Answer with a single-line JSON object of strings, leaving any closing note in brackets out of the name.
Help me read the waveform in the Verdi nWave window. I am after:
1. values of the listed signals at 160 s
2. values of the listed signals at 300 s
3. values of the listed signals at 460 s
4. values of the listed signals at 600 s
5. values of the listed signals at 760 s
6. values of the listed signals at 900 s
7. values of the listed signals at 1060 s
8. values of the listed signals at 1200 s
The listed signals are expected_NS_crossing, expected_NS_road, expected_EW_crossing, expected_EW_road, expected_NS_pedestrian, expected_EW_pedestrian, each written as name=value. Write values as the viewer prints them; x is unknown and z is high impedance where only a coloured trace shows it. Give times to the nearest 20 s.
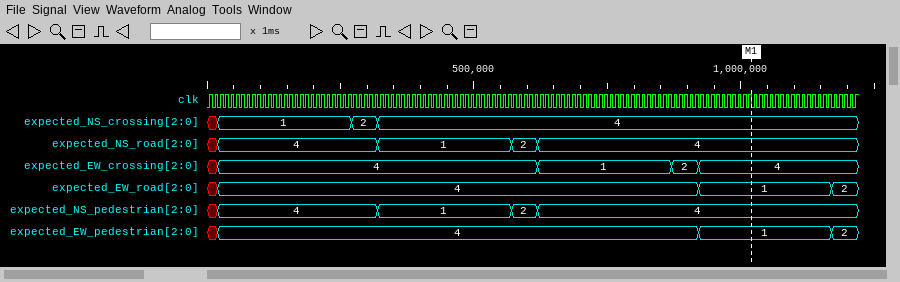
{"values of the listed signals at 160 s": "expected_NS_crossing=1, expected_NS_road=4, expected_EW_crossing=4, expected_EW_road=4, expected_NS_pedestrian=4, expected_EW_pedestrian=4", "values of the listed signals at 300 s": "expected_NS_crossing=2, expected_NS_road=4, expected_EW_crossing=4, expected_EW_road=4, expected_NS_pedestrian=4, expected_EW_pedestrian=4", "values of the listed signals at 460 s": "expected_NS_crossing=4, expected_NS_road=1, expected_EW_crossing=4, expected_EW_road=4, expected_NS_pedestrian=1, expected_EW_pedestrian=4", "values of the listed signals at 600 s": "expected_NS_crossing=4, expected_NS_road=2, expected_EW_crossing=4, expected_EW_road=4, expected_NS_pedestrian=2, expected_EW_pedestrian=4", "values of the listed signals at 760 s": "expected_NS_crossing=4, expected_NS_road=4, expected_EW_crossing=1, expected_EW_road=4, expected_NS_pedestrian=4, expected_EW_pedestrian=4", "values of the listed signals at 900 s": "expected_NS_crossing=4, expected_NS_road=4, expected_EW_crossing=2, expected_EW_road=4, expected_NS_pedestrian=4, expected_EW_pedestrian=4", "values of the listed signals at 1060 s": "expected_NS_crossing=4, expected_NS_road=4, expected_EW_crossing=4, expected_EW_road=1, expected_NS_pedestrian=4, expected_EW_pedestrian=1", "values of the listed signals at 1200 s": "expected_NS_crossing=4, expected_NS_road=4, expected_EW_crossing=4, expected_EW_road=2, expected_NS_pedestrian=4, expected_EW_pedestrian=2"}
